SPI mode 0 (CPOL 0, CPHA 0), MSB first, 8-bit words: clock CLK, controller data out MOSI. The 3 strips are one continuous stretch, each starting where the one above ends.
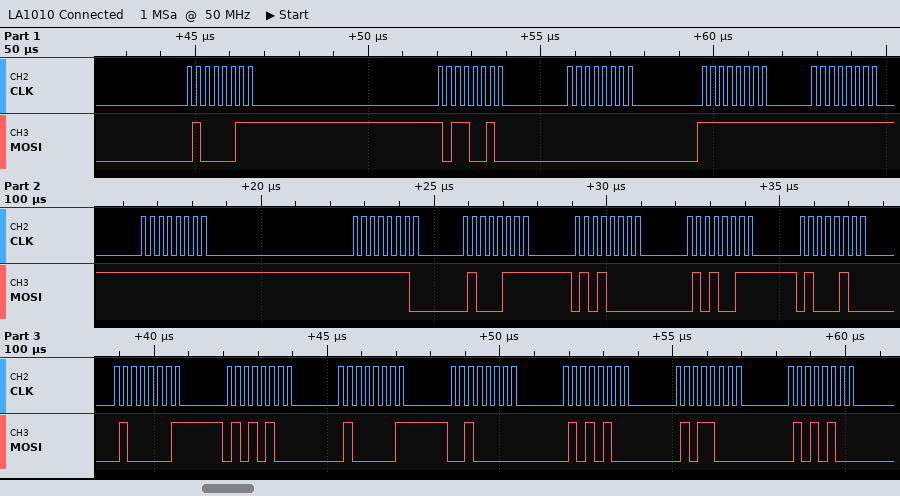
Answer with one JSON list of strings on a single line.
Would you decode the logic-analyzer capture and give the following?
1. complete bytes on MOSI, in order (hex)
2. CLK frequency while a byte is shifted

["43 B2 00 FF FF FF FE 47 50 53 44 41 54 41 20 54 58 54", "4 MHz"]
